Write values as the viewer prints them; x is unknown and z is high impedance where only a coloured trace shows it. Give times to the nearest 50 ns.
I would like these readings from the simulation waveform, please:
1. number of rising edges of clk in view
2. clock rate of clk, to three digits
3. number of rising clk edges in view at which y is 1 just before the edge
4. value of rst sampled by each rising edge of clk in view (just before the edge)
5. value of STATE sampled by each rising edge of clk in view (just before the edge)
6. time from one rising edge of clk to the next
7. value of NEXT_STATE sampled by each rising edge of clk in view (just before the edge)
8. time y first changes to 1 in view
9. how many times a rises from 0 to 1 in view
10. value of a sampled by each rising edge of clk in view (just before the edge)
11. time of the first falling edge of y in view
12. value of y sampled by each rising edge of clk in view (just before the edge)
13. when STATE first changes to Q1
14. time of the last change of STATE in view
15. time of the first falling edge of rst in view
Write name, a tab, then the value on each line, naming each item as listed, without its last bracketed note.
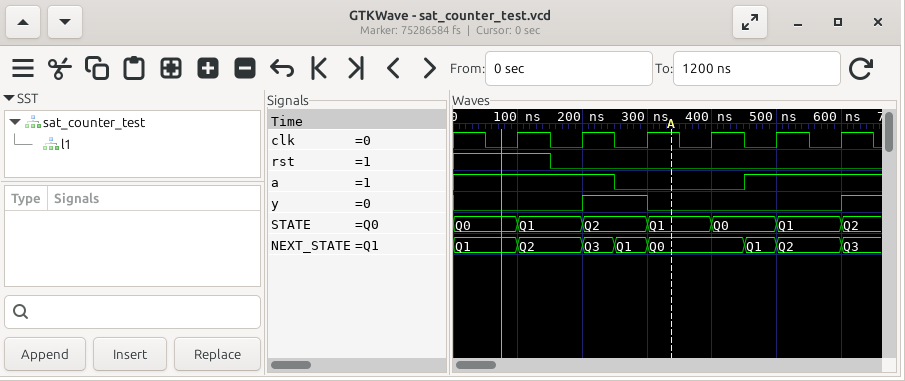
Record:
number of rising edges of clk in view	6
clock rate of clk, to three digits	10.0 MHz
number of rising clk edges in view at which y is 1 just before the edge	1
value of rst sampled by each rising edge of clk in view	1 0 0 0 0 0
value of STATE sampled by each rising edge of clk in view	Q0, Q1, Q2, Q1, Q0, Q1
time from one rising edge of clk to the next	100 ns
value of NEXT_STATE sampled by each rising edge of clk in view	Q1, Q2, Q1, Q0, Q1, Q2
time y first changes to 1 in view	200 ns
how many times a rises from 0 to 1 in view	1
value of a sampled by each rising edge of clk in view	1 1 0 0 1 1
time of the first falling edge of y in view	300 ns
value of y sampled by each rising edge of clk in view	0 0 1 0 0 0
when STATE first changes to Q1	100 ns
time of the last change of STATE in view	600 ns
time of the first falling edge of rst in view	150 ns
